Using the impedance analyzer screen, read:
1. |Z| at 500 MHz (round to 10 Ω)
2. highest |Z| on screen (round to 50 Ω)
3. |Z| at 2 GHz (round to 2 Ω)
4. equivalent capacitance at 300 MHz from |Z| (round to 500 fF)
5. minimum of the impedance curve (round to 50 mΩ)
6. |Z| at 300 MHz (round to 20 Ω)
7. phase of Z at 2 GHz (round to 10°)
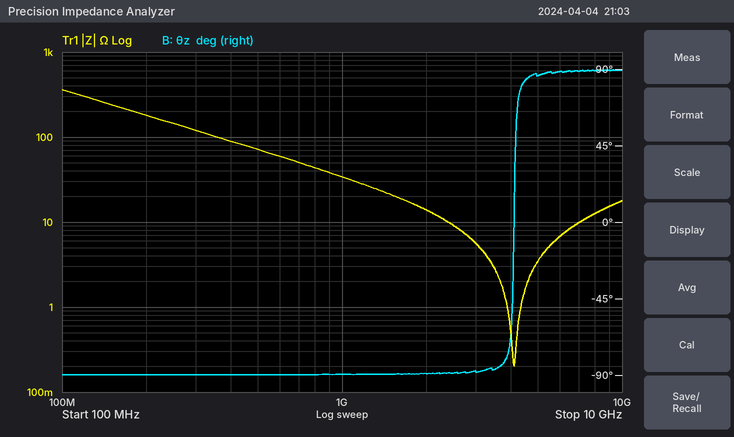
70 Ω
350 Ω
14 Ω
4.5 pF
200 mΩ
120 Ω
-90°
